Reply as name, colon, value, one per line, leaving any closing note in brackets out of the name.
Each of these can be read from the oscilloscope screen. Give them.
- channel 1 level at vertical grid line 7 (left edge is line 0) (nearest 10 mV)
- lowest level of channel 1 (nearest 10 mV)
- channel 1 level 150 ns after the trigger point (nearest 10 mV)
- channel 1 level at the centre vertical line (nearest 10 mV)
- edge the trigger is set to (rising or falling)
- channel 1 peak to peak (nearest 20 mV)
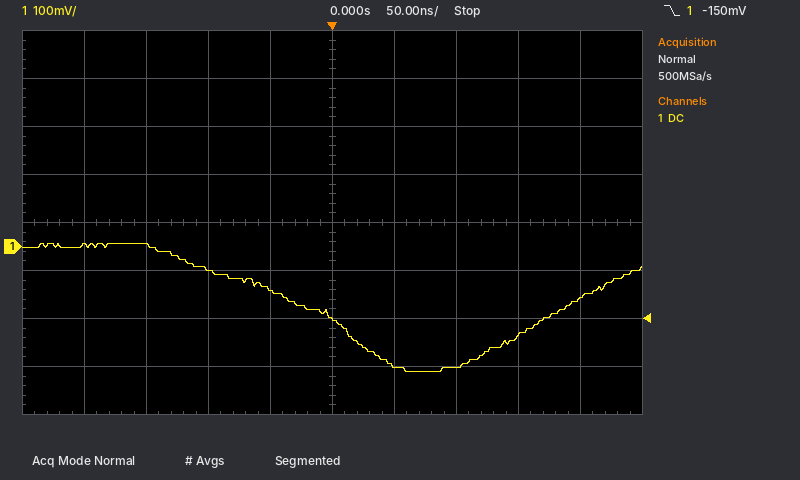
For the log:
channel 1 level at vertical grid line 7 (left edge is line 0): -250 mV
lowest level of channel 1: -260 mV
channel 1 level 150 ns after the trigger point: -190 mV
channel 1 level at the centre vertical line: -150 mV
edge the trigger is set to: falling
channel 1 peak to peak: 260 mV
